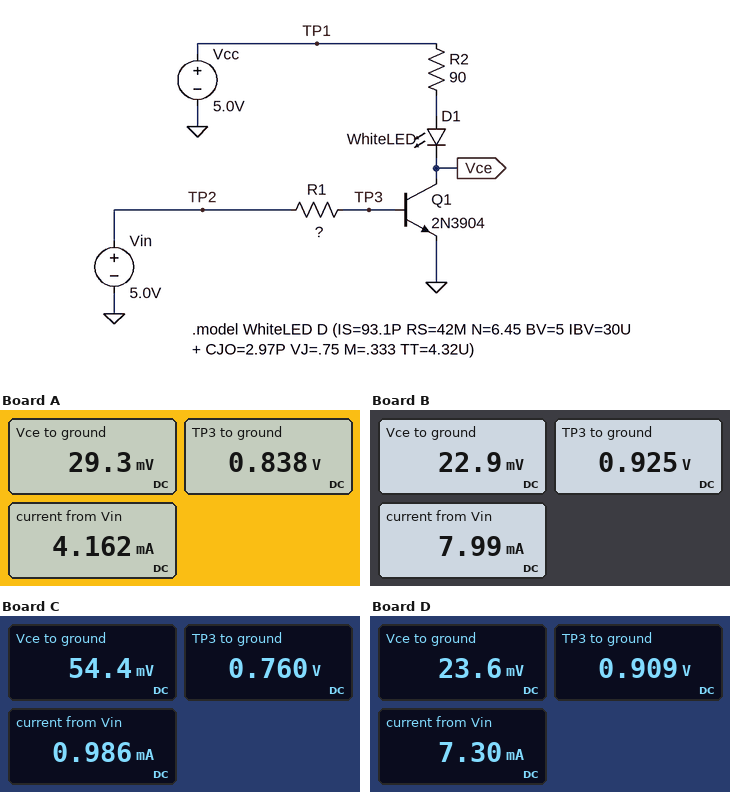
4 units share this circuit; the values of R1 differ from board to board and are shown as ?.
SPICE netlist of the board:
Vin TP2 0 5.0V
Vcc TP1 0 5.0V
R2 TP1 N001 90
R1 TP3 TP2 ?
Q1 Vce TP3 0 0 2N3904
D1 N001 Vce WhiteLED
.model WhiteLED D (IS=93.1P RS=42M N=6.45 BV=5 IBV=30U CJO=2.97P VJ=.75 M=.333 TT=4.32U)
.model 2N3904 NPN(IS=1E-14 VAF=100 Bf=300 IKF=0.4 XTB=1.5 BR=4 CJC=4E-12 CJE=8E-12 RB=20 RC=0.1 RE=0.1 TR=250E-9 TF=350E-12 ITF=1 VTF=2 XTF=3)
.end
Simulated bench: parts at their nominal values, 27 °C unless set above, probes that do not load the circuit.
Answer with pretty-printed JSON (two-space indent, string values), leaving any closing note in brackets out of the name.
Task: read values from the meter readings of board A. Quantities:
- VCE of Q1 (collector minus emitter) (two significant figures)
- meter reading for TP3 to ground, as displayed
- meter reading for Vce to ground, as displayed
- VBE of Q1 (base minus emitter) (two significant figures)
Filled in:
{
  "VCE of Q1 (collector minus emitter)": "29 mV",
  "meter reading for TP3 to ground, as displayed": "0.838 V",
  "meter reading for Vce to ground, as displayed": "29.3 mV",
  "VBE of Q1 (base minus emitter)": "840 mV"
}
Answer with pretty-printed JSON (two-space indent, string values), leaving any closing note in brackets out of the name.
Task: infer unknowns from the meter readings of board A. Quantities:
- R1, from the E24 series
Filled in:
{
  "R1, from the E24 series": "1 kΩ"
}
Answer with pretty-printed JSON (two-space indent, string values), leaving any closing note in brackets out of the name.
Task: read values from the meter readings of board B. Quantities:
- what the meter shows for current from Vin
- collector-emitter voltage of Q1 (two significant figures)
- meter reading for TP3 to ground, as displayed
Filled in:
{
  "what the meter shows for current from Vin": "7.99 mA",
  "collector-emitter voltage of Q1": "23 mV",
  "meter reading for TP3 to ground, as displayed": "0.925 V"
}
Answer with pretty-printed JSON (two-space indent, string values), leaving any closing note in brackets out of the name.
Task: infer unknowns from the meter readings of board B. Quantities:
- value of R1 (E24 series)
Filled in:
{
  "value of R1": "510 Ω"
}
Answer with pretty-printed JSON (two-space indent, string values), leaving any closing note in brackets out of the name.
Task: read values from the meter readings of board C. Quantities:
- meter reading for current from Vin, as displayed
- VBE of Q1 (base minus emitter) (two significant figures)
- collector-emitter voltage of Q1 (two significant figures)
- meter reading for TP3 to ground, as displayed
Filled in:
{
  "meter reading for current from Vin, as displayed": "0.986 mA",
  "VBE of Q1 (base minus emitter)": "760 mV",
  "collector-emitter voltage of Q1": "54 mV",
  "meter reading for TP3 to ground, as displayed": "0.760 V"
}
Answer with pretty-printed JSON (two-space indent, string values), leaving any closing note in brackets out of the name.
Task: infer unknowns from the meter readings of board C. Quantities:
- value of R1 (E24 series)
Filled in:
{
  "value of R1": "4.3 kΩ"
}
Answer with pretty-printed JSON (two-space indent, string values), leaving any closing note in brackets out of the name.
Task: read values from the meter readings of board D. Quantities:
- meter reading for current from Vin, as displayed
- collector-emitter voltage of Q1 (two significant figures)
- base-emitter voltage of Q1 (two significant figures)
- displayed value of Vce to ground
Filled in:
{
  "meter reading for current from Vin, as displayed": "7.30 mA",
  "collector-emitter voltage of Q1": "24 mV",
  "base-emitter voltage of Q1": "910 mV",
  "displayed value of Vce to ground": "23.6 mV"
}
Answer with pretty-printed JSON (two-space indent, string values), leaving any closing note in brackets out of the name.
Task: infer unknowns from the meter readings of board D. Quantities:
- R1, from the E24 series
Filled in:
{
  "R1, from the E24 series": "560 Ω"
}
